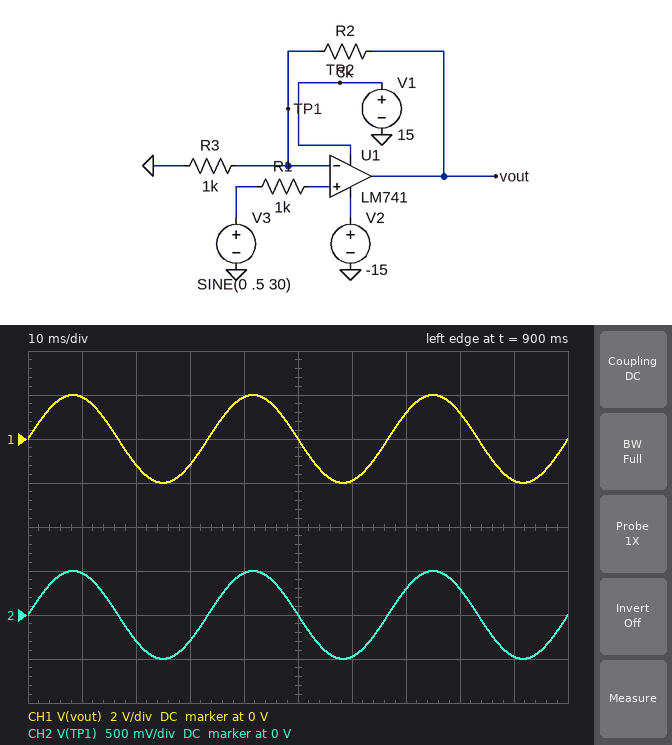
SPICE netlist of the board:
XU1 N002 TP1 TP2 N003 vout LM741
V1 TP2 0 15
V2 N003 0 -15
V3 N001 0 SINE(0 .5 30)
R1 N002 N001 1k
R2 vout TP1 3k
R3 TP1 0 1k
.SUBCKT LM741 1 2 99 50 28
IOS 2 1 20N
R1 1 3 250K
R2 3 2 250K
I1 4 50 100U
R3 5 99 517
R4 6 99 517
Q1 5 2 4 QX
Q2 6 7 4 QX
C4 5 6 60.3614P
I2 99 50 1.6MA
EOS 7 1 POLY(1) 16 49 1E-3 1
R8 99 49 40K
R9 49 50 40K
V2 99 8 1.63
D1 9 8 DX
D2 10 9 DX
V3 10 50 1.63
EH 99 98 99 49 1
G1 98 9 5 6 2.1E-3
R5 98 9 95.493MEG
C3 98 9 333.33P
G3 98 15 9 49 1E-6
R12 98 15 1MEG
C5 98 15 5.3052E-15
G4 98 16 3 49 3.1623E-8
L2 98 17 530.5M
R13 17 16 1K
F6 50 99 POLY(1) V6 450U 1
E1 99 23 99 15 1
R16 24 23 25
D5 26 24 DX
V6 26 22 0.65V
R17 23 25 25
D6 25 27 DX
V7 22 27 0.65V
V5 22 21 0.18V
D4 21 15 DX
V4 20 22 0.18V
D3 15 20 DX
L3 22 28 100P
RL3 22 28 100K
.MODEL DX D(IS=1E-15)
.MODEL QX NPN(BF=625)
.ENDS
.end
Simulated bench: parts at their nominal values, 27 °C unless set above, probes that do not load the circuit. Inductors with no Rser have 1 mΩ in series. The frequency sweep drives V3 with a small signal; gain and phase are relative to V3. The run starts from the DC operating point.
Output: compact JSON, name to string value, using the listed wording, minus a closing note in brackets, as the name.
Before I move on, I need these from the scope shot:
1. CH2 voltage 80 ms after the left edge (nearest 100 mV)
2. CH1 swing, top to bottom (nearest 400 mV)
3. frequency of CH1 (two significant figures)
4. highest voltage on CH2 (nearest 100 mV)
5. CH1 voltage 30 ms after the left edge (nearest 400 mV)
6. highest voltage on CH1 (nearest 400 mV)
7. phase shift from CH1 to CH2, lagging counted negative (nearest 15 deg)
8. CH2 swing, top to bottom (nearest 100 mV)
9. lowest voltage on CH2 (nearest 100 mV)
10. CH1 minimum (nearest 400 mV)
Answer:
{"CH2 voltage 80 ms after the left edge": "300 mV", "CH1 swing, top to bottom": "4.0 V", "frequency of CH1": "30 Hz", "highest voltage on CH2": "500 mV", "CH1 voltage 30 ms after the left edge": "-1.2 V", "highest voltage on CH1": "2.0 V", "phase shift from CH1 to CH2, lagging counted negative": "0 deg", "CH2 swing, top to bottom": "1.0 V", "lowest voltage on CH2": "-500 mV", "CH1 minimum": "-2.0 V"}
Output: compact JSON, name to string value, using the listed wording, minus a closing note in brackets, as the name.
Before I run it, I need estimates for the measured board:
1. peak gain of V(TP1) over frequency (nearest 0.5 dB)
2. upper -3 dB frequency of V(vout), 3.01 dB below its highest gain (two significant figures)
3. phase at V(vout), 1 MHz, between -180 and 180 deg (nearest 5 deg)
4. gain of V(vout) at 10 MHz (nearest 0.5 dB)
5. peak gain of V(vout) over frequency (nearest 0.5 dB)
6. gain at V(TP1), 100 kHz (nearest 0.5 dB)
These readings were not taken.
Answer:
{"peak gain of V(TP1) over frequency": "0 dB", "upper -3 dB frequency of V(vout), 3.01 dB below its highest gain": "270 kHz", "phase at V(vout), 1 MHz, between -180 and 180 deg": "-100 deg", "gain of V(vout) at 10 MHz": "-32.0 dB", "peak gain of V(vout) over frequency": "12.0 dB", "gain at V(TP1), 100 kHz": "-0.5 dB"}
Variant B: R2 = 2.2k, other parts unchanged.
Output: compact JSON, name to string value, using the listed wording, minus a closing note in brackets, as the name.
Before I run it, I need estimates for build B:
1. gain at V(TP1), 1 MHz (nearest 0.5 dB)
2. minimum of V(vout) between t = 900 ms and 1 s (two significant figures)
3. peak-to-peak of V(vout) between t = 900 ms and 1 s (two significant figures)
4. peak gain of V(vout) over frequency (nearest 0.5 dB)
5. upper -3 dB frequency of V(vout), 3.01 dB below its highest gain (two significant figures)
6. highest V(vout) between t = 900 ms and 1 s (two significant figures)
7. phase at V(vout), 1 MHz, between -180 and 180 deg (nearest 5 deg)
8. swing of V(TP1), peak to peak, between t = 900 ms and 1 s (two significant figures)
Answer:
{"gain at V(TP1), 1 MHz": "-10.5 dB", "minimum of V(vout) between t = 900 ms and 1 s": "-1.6 V", "peak-to-peak of V(vout) between t = 900 ms and 1 s": "3.2 V", "peak gain of V(vout) over frequency": "10.0 dB", "upper -3 dB frequency of V(vout), 3.01 dB below its highest gain": "340 kHz", "highest V(vout) between t = 900 ms and 1 s": "1.6 V", "phase at V(vout), 1 MHz, between -180 and 180 deg": "-95 deg", "swing of V(TP1), peak to peak, between t = 900 ms and 1 s": "1.0 V"}
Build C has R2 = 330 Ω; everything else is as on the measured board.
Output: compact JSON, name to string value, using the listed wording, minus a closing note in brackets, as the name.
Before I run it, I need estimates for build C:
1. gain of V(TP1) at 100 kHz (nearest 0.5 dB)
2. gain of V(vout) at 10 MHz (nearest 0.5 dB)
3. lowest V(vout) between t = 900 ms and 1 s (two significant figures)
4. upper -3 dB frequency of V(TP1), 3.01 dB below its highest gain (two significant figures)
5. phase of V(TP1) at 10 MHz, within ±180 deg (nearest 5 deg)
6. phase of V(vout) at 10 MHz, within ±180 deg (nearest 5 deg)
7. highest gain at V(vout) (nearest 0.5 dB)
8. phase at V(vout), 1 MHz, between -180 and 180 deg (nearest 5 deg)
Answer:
{"gain of V(TP1) at 100 kHz": "0 dB", "gain of V(vout) at 10 MHz": "-32.5 dB", "lowest V(vout) between t = 900 ms and 1 s": "-660 mV", "upper -3 dB frequency of V(TP1), 3.01 dB below its highest gain": "930 kHz", "phase of V(TP1) at 10 MHz, within ±180 deg": "-155 deg", "phase of V(vout) at 10 MHz, within ±180 deg": "-155 deg", "highest gain at V(vout)": "2.5 dB", "phase at V(vout), 1 MHz, between -180 and 180 deg": "-75 deg"}
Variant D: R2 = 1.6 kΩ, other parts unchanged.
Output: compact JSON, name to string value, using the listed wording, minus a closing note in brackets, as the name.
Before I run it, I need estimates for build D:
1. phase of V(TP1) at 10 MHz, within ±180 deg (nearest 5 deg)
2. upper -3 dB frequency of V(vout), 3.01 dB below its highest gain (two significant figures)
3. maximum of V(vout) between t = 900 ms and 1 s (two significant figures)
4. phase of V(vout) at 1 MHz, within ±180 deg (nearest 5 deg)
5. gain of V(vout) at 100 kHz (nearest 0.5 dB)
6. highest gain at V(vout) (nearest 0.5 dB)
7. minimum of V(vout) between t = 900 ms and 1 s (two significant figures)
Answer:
{"phase of V(TP1) at 10 MHz, within ±180 deg": "-155 deg", "upper -3 dB frequency of V(vout), 3.01 dB below its highest gain": "430 kHz", "maximum of V(vout) between t = 900 ms and 1 s": "1.3 V", "phase of V(vout) at 1 MHz, within ±180 deg": "-90 deg", "gain of V(vout) at 100 kHz": "8.0 dB", "highest gain at V(vout)": "8.5 dB", "minimum of V(vout) between t = 900 ms and 1 s": "-1.3 V"}
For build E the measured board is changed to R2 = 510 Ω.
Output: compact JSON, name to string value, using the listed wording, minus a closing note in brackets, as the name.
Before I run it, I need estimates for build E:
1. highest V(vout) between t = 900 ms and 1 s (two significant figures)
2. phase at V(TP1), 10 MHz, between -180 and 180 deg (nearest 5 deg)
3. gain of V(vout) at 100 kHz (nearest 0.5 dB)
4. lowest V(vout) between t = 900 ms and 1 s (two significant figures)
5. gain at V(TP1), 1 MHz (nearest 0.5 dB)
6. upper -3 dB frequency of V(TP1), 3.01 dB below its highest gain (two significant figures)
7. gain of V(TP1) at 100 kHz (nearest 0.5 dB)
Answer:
{"highest V(vout) between t = 900 ms and 1 s": "760 mV", "phase at V(TP1), 10 MHz, between -180 and 180 deg": "-155 deg", "gain of V(vout) at 100 kHz": "3.5 dB", "lowest V(vout) between t = 900 ms and 1 s": "-750 mV", "gain at V(TP1), 1 MHz": "-4.5 dB", "upper -3 dB frequency of V(TP1), 3.01 dB below its highest gain": "800 kHz", "gain of V(TP1) at 100 kHz": "0 dB"}
